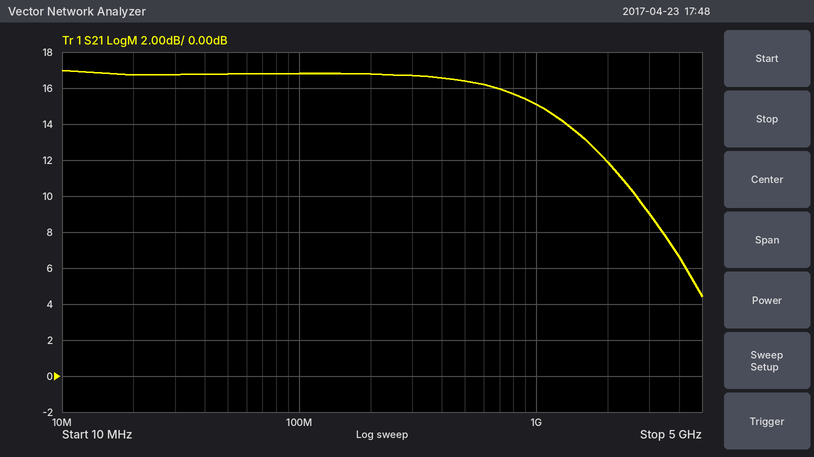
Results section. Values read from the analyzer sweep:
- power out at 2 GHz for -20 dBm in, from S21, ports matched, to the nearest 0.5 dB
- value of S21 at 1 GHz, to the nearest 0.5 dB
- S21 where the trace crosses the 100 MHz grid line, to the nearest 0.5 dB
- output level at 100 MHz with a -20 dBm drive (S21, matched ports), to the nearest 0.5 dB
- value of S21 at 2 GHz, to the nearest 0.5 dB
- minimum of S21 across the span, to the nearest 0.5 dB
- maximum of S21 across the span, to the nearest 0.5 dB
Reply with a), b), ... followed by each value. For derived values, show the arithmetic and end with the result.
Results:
a) -20 dBm + (12.0 dB) = -8.0 dBm
b) 15.0 dB
c) 17.0 dB
d) -20 dBm + (17.0 dB) = -3.0 dBm
e) 12.0 dB
f) 4.5 dB
g) 17.0 dB
